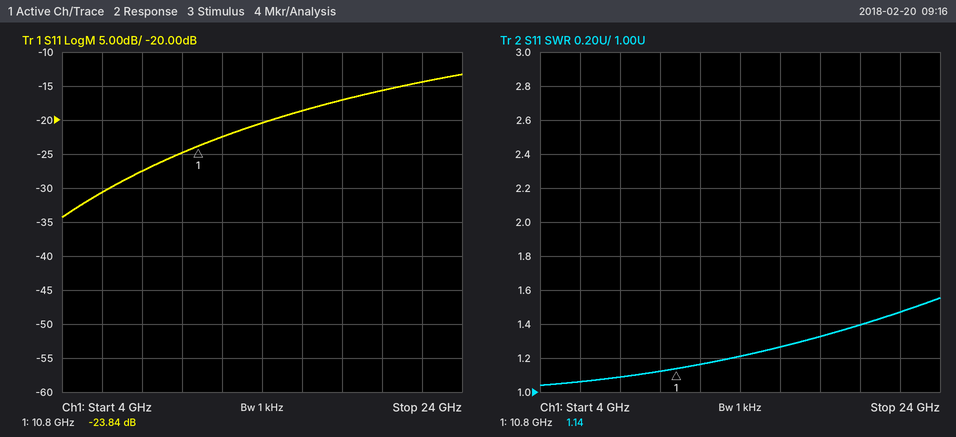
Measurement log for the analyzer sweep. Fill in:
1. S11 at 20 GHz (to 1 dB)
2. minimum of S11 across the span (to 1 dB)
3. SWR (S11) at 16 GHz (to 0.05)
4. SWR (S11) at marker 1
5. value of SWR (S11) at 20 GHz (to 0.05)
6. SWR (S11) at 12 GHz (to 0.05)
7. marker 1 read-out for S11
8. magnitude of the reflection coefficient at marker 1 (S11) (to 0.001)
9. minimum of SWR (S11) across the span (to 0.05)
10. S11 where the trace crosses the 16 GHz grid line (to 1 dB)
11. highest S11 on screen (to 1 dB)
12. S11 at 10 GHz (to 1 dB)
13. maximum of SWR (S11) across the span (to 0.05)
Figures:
-16 dB
-34 dB
1.25
1.14
1.40
1.15
-23.84 dB
0.064
1.05
-19 dB
-13 dB
-25 dB
1.55
